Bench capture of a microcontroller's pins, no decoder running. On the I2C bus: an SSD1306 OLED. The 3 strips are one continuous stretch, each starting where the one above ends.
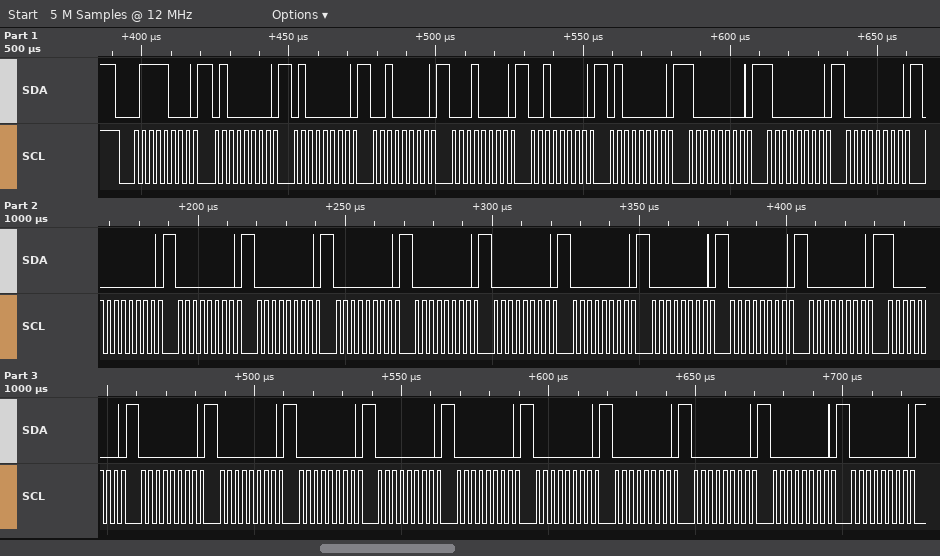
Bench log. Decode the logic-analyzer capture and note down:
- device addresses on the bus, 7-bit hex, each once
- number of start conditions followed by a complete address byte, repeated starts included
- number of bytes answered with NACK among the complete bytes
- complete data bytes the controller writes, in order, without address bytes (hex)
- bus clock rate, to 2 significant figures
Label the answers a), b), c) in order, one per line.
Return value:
a) 0x3C
b) 1
c) 0
d) 40 40 20 10 20 40 80 80 00 00 00 00 00 00 00 00 00 00 00 80 00 00 00 00 00 00 00 00 00 00
e) 400 kHz
